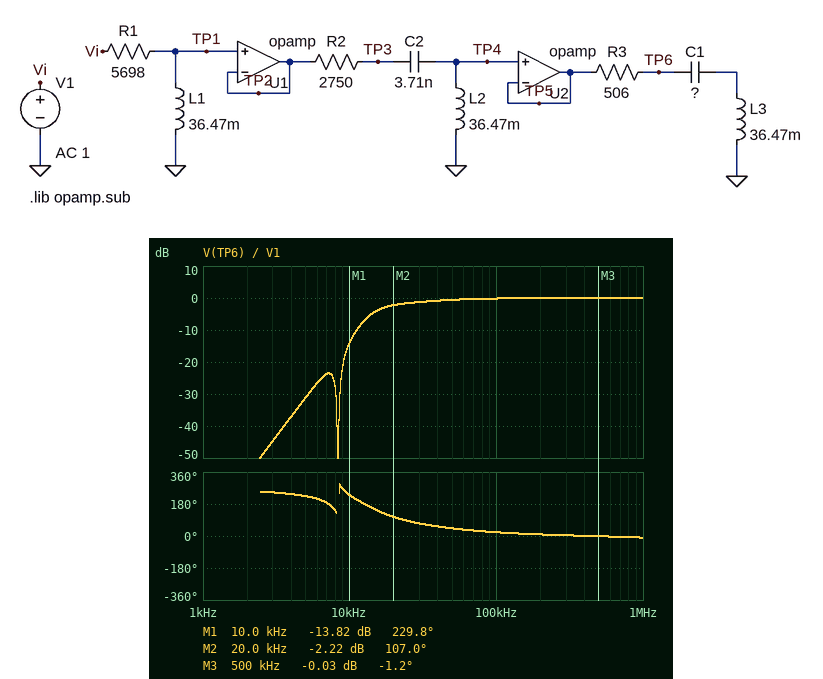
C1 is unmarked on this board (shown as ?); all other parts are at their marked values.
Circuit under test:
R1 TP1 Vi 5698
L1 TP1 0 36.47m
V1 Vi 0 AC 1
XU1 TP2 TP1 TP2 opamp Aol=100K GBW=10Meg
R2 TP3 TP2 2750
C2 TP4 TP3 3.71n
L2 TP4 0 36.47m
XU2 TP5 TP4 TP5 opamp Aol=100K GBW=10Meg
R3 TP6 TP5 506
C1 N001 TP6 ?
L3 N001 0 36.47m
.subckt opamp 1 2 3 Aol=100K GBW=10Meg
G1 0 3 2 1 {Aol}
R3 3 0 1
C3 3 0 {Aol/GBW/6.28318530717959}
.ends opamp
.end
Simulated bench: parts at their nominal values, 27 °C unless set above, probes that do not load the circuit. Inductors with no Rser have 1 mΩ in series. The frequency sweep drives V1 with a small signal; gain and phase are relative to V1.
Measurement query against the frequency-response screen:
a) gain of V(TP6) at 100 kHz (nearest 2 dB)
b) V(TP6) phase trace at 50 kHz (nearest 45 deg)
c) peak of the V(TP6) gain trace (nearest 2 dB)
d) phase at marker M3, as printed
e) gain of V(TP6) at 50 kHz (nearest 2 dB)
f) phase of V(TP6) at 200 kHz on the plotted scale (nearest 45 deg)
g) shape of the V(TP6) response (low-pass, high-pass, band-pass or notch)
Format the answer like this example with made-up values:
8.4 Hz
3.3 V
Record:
0 dB
45 deg
0 dB
-1.2 deg
0 dB
0 deg
high-pass
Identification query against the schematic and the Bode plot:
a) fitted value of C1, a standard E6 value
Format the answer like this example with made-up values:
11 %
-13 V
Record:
10 nF
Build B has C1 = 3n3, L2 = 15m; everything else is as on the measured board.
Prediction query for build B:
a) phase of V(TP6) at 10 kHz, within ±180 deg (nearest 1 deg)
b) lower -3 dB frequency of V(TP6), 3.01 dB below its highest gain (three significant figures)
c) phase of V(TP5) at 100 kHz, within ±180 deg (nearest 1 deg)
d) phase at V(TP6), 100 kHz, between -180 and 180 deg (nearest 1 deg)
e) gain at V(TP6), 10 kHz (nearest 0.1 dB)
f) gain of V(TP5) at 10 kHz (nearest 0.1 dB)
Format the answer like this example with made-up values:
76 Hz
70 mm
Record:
-163 deg
30.1 kHz
30 deg
31 deg
-22.0 dB
-21.8 dB
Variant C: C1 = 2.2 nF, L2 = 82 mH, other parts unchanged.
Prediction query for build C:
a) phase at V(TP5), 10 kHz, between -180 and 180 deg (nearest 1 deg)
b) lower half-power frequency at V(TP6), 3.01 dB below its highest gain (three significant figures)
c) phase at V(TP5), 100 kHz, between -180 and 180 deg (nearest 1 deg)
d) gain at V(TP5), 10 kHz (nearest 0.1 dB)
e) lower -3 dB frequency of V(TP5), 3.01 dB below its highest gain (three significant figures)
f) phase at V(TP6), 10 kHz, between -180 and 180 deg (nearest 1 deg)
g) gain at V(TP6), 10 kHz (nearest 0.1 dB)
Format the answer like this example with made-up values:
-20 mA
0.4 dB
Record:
141 deg
20.8 kHz
16 deg
-3.5 dB
11.3 kHz
135 deg
-3.6 dB
